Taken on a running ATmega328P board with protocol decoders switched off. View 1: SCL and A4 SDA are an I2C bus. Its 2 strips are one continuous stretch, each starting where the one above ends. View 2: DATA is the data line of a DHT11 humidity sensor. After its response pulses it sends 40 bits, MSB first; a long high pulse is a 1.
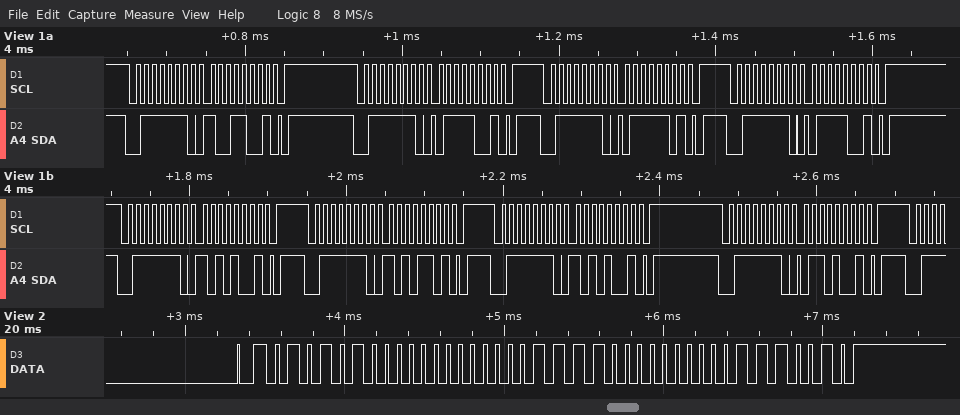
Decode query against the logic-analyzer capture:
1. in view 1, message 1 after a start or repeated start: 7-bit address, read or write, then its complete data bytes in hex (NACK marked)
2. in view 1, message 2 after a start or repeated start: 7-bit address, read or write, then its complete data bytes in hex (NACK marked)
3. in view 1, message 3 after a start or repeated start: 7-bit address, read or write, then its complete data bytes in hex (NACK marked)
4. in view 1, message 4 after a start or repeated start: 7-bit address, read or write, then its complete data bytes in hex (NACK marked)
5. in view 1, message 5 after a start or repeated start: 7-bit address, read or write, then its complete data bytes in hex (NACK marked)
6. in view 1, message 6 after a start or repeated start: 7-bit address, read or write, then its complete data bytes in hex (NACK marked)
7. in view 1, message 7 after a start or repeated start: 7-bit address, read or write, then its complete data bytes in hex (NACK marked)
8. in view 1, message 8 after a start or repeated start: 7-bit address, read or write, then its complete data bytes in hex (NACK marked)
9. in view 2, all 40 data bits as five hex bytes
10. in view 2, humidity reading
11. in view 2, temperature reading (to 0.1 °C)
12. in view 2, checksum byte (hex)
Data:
0x3F write: 99
0x3F write: 79
0x3F write: 7D
0x3F write: 79
0x3F write: A9
0x3F write: AD
0x3F write: A9
0x3F write: 69
54 00 1E 00 72
84 %
30.0 °C
0x72
